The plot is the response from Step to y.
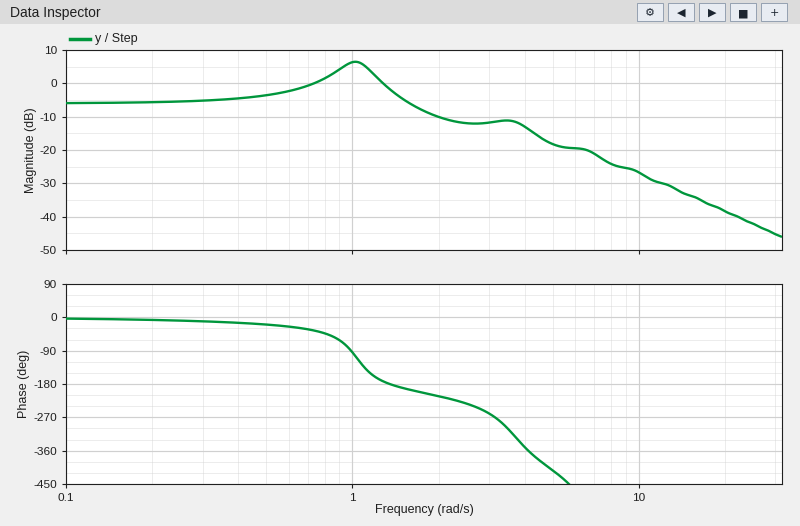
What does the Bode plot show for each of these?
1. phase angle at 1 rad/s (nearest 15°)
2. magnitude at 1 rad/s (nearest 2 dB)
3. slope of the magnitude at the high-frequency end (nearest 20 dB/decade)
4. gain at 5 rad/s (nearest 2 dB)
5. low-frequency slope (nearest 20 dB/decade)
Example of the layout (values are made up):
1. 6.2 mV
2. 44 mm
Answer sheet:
1. -90°
2. 6 dB
3. -40 dB/decade
4. -18 dB
5. 0 dB/decade
